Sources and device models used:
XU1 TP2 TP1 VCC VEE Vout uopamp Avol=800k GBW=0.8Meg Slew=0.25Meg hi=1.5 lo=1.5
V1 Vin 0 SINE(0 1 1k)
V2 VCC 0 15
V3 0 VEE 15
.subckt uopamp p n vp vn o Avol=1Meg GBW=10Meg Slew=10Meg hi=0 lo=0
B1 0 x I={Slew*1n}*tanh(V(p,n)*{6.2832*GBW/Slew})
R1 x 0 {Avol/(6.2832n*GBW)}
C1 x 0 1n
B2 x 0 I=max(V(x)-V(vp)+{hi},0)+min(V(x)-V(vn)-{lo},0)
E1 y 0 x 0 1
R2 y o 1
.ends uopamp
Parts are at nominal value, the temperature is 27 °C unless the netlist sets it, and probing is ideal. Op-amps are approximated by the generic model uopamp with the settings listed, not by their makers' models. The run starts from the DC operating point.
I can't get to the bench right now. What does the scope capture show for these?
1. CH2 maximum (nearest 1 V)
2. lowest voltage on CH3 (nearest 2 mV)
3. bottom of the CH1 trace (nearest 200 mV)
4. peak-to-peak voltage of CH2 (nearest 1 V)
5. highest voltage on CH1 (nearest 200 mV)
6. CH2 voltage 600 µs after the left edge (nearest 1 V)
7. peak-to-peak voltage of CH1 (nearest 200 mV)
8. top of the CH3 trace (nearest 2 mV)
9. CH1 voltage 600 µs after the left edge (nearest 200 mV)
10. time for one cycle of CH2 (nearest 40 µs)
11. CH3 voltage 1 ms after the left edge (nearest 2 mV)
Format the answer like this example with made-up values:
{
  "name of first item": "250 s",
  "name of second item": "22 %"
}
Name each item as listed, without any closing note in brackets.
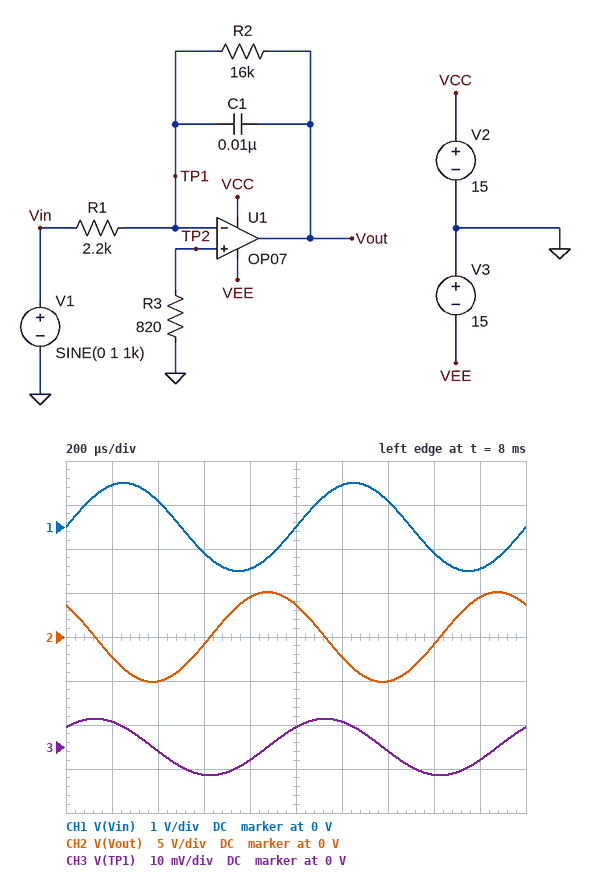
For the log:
{
  "CH2 maximum": "5 V",
  "lowest voltage on CH3": "-6 mV",
  "bottom of the CH1 trace": "-1.0 V",
  "peak-to-peak voltage of CH2": "10 V",
  "highest voltage on CH1": "1.0 V",
  "CH2 voltage 600 µs after the left edge": "-1 V",
  "peak-to-peak voltage of CH1": "2.0 V",
  "top of the CH3 trace": "6 mV",
  "CH1 voltage 600 µs after the left edge": "-600 mV",
  "time for one cycle of CH2": "1.00 ms",
  "CH3 voltage 1 ms after the left edge": "4 mV"
}
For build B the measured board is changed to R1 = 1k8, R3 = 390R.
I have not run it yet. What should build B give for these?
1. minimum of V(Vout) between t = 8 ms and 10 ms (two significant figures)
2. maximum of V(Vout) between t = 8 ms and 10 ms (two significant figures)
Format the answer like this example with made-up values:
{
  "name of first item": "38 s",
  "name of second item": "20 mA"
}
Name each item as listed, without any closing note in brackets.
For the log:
{
  "minimum of V(Vout) between t = 8 ms and 10 ms": "-6.2 V",
  "maximum of V(Vout) between t = 8 ms and 10 ms": "6.2 V"
}
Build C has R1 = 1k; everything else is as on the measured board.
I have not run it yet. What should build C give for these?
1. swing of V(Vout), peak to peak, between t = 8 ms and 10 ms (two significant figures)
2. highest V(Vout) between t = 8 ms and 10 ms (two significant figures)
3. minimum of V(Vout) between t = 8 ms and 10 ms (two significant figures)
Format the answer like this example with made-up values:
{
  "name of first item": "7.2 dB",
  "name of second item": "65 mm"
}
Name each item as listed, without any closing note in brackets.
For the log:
{
  "swing of V(Vout), peak to peak, between t = 8 ms and 10 ms": "22 V",
  "highest V(Vout) between t = 8 ms and 10 ms": "11 V",
  "minimum of V(Vout) between t = 8 ms and 10 ms": "-11 V"
}
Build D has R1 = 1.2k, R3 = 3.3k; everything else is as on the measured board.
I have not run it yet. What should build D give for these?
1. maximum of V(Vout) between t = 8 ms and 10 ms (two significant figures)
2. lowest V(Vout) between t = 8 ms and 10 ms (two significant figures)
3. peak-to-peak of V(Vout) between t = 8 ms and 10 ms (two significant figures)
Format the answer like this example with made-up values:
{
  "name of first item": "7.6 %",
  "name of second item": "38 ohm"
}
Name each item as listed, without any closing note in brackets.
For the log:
{
  "maximum of V(Vout) between t = 8 ms and 10 ms": "9.3 V",
  "lowest V(Vout) between t = 8 ms and 10 ms": "-9.3 V",
  "peak-to-peak of V(Vout) between t = 8 ms and 10 ms": "19 V"
}
